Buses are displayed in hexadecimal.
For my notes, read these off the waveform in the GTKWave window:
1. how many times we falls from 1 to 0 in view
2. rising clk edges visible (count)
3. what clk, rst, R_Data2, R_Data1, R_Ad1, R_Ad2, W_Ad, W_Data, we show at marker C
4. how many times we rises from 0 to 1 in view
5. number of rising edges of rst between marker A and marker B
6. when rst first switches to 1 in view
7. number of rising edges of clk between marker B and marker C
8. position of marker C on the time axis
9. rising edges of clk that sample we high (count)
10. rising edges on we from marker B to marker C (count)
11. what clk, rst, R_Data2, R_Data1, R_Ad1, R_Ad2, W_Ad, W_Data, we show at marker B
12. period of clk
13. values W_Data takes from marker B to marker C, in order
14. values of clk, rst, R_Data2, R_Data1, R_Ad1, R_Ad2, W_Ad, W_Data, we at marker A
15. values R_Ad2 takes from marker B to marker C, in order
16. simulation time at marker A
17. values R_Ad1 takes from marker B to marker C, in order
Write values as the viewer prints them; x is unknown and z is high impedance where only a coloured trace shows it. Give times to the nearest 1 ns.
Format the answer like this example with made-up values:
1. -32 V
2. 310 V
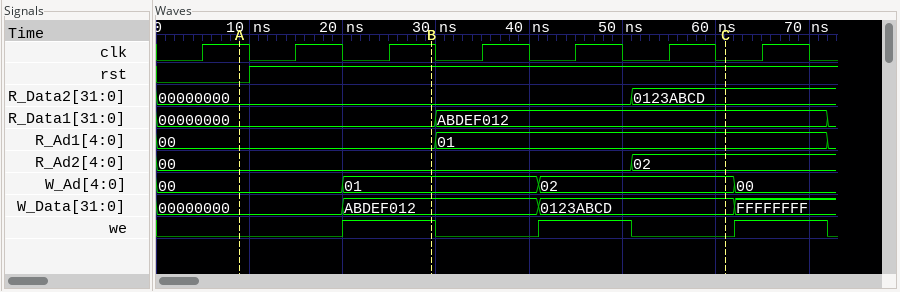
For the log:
1. 3
2. 7
3. clk=0, rst=1, R_Data2=0123ABCD, R_Data1=ABDEF012, R_Ad1=01, R_Ad2=02, W_Ad=02, W_Data=0123ABCD, we=0
4. 3
5. 1
6. 10 ns
7. 3
8. 61 ns
9. 3
10. 1
11. clk=1, rst=1, R_Data2=00000000, R_Data1=00000000, R_Ad1=00, R_Ad2=00, W_Ad=01, W_Data=ABDEF012, we=1
12. 10 ns
13. ABDEF012, 0123ABCD
14. clk=1, rst=0, R_Data2=00000000, R_Data1=00000000, R_Ad1=00, R_Ad2=00, W_Ad=00, W_Data=00000000, we=0
15. 00, 02
16. 9 ns
17. 00, 01
